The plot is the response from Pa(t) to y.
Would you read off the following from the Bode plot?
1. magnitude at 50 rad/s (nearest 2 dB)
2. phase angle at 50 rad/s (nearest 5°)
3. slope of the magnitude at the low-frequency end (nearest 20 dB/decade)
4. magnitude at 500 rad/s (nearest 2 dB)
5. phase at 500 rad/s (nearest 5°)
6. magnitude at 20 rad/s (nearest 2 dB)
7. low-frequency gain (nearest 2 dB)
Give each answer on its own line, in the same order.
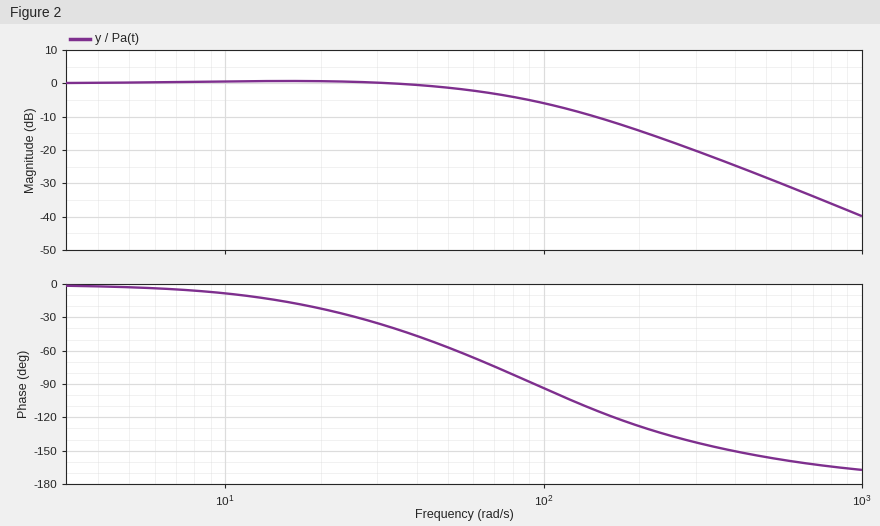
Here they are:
-2 dB
-55°
0 dB/decade
-28 dB
-155°
0 dB
0 dB
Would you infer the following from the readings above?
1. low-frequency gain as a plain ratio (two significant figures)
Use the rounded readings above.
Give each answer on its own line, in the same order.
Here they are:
1.0
